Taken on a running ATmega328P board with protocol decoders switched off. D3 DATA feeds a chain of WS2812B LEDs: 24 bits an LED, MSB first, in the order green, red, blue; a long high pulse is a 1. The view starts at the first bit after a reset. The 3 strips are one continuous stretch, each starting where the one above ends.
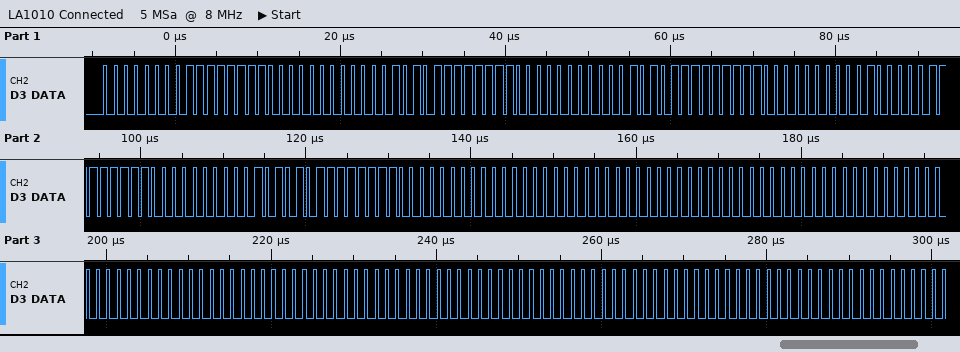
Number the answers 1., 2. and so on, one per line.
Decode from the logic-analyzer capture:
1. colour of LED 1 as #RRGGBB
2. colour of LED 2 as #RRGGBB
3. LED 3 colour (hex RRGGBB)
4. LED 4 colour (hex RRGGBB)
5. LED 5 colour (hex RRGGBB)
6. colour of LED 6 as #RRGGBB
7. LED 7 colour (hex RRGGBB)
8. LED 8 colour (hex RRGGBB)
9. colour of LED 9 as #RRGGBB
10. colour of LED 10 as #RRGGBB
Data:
1. #FF0000
2. #FF0A00
3. #FF1500
4. #FF2000
5. #FF2A00
6. #000000
7. #000000
8. #000000
9. #000000
10. #000000
